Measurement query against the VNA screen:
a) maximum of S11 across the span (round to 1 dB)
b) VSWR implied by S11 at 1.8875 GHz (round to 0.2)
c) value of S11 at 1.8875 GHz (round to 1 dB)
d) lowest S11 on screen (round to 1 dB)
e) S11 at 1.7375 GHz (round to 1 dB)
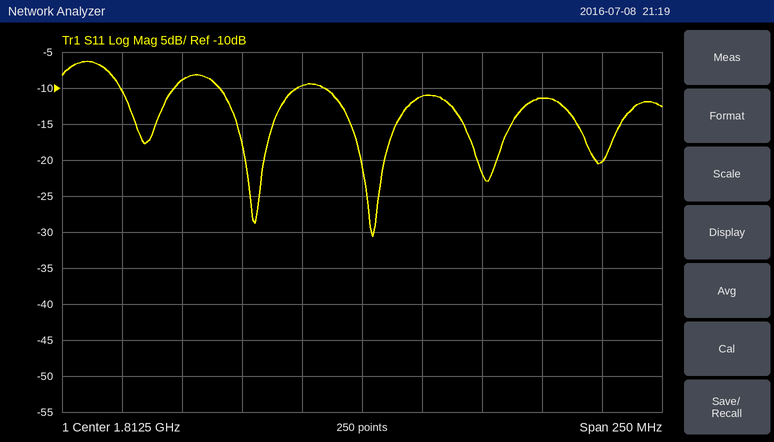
-6 dB
1.8
-11 dB
-31 dB
-9 dB
